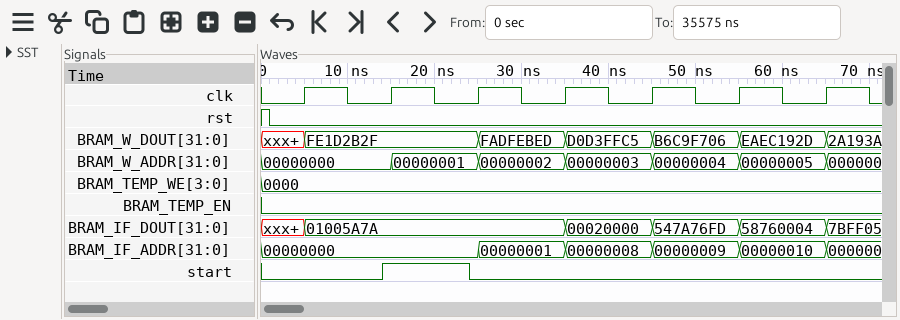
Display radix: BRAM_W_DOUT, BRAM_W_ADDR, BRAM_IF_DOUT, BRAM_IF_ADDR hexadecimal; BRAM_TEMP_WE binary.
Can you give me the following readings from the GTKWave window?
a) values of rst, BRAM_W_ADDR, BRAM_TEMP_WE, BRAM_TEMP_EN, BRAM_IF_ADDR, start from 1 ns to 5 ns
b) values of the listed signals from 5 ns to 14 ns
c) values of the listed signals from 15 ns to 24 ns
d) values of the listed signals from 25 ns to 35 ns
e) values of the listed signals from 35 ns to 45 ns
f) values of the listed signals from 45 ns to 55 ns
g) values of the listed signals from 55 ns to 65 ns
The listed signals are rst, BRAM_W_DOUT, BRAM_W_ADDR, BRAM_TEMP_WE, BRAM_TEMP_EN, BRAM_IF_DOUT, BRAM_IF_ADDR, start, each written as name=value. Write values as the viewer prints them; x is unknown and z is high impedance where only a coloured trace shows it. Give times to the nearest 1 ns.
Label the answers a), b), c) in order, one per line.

a) rst=0, BRAM_W_ADDR=00000000, BRAM_TEMP_WE=0000, BRAM_TEMP_EN=0, BRAM_IF_ADDR=00000000, start=0
b) rst=0, BRAM_W_DOUT=FE1D2B2F, BRAM_W_ADDR=00000000, BRAM_TEMP_WE=0000, BRAM_TEMP_EN=0, BRAM_IF_DOUT=01005A7A, BRAM_IF_ADDR=00000000, start=0
c) rst=0, BRAM_W_DOUT=FE1D2B2F, BRAM_W_ADDR=00000001, BRAM_TEMP_WE=0000, BRAM_TEMP_EN=0, BRAM_IF_DOUT=01005A7A, BRAM_IF_ADDR=00000000, start=1
d) rst=0, BRAM_W_DOUT=FADFEBED, BRAM_W_ADDR=00000002, BRAM_TEMP_WE=0000, BRAM_TEMP_EN=0, BRAM_IF_DOUT=01005A7A, BRAM_IF_ADDR=00000001, start=0
e) rst=0, BRAM_W_DOUT=D0D3FFC5, BRAM_W_ADDR=00000003, BRAM_TEMP_WE=0000, BRAM_TEMP_EN=0, BRAM_IF_DOUT=00020000, BRAM_IF_ADDR=00000008, start=0
f) rst=0, BRAM_W_DOUT=B6C9F706, BRAM_W_ADDR=00000004, BRAM_TEMP_WE=0000, BRAM_TEMP_EN=0, BRAM_IF_DOUT=547A76FD, BRAM_IF_ADDR=00000009, start=0
g) rst=0, BRAM_W_DOUT=EAEC192D, BRAM_W_ADDR=00000005, BRAM_TEMP_WE=0000, BRAM_TEMP_EN=0, BRAM_IF_DOUT=58760004, BRAM_IF_ADDR=00000010, start=0
